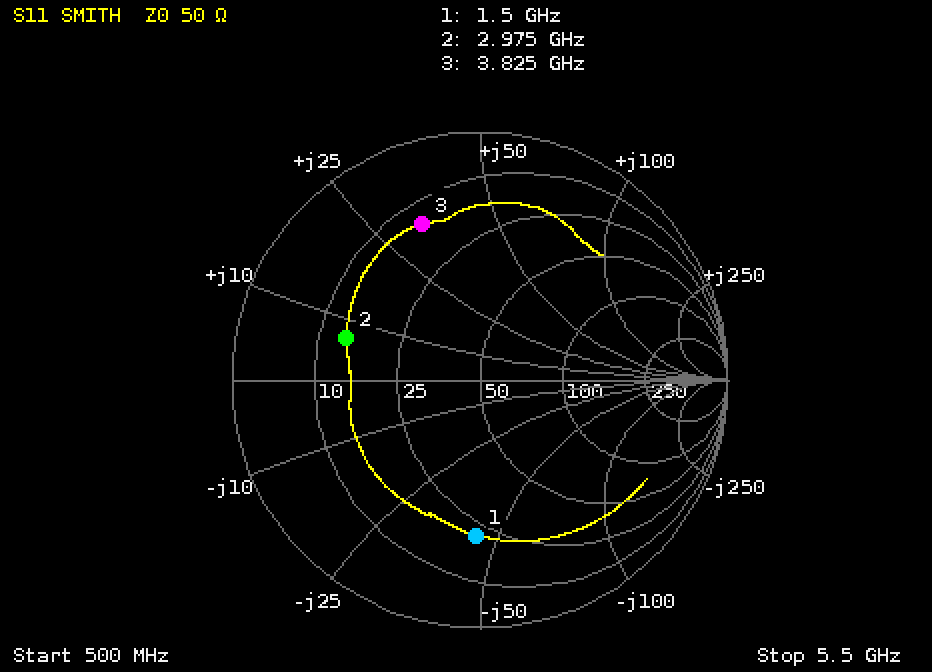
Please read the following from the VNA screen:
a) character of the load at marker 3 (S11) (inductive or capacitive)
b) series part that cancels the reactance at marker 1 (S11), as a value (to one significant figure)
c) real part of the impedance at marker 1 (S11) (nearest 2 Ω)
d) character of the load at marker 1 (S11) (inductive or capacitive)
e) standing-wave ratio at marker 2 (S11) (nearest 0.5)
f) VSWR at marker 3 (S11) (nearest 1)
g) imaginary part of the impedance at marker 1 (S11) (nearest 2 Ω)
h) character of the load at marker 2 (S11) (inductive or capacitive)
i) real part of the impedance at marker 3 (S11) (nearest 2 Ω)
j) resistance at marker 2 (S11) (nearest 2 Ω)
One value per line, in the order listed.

inductive
5 nH
22 Ω
capacitive
3.5
5
-44 Ω
inductive
14 Ω
14 Ω
